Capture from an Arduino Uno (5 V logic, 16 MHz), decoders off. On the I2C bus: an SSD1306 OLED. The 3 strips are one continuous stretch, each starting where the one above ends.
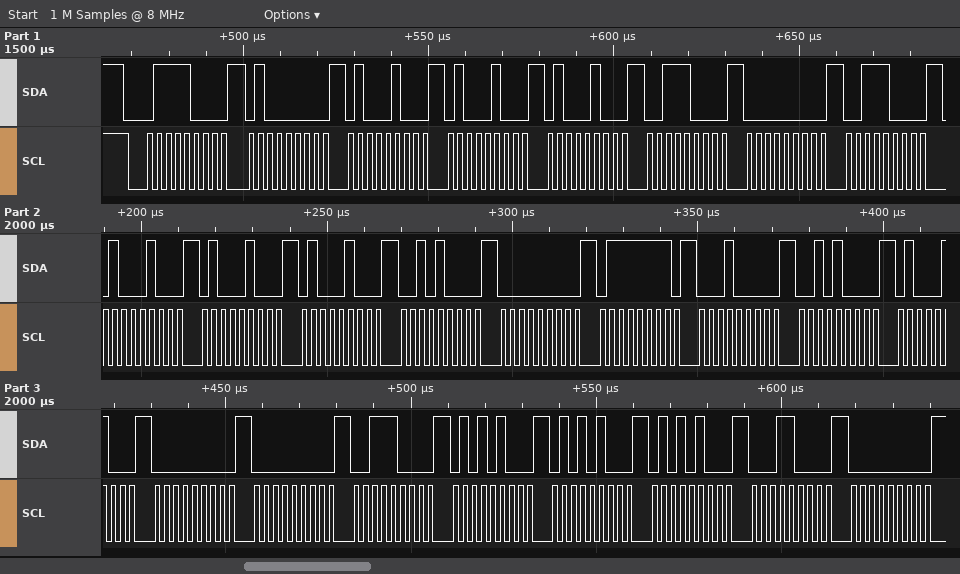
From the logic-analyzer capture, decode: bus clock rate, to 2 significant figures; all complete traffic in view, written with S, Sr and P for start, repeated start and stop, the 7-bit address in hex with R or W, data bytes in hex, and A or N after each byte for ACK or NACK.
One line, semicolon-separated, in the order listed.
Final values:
400 kHz; S 3CW A 40 A 44 A 44 A 44 A 38 A 00 A 38 A 44 A 44 A 44 A 28 A 00 A 7F A 10 A 28 A 44 A 00 A 00 A 38 A 54 A 54 A 54 A 18 A 00 A
